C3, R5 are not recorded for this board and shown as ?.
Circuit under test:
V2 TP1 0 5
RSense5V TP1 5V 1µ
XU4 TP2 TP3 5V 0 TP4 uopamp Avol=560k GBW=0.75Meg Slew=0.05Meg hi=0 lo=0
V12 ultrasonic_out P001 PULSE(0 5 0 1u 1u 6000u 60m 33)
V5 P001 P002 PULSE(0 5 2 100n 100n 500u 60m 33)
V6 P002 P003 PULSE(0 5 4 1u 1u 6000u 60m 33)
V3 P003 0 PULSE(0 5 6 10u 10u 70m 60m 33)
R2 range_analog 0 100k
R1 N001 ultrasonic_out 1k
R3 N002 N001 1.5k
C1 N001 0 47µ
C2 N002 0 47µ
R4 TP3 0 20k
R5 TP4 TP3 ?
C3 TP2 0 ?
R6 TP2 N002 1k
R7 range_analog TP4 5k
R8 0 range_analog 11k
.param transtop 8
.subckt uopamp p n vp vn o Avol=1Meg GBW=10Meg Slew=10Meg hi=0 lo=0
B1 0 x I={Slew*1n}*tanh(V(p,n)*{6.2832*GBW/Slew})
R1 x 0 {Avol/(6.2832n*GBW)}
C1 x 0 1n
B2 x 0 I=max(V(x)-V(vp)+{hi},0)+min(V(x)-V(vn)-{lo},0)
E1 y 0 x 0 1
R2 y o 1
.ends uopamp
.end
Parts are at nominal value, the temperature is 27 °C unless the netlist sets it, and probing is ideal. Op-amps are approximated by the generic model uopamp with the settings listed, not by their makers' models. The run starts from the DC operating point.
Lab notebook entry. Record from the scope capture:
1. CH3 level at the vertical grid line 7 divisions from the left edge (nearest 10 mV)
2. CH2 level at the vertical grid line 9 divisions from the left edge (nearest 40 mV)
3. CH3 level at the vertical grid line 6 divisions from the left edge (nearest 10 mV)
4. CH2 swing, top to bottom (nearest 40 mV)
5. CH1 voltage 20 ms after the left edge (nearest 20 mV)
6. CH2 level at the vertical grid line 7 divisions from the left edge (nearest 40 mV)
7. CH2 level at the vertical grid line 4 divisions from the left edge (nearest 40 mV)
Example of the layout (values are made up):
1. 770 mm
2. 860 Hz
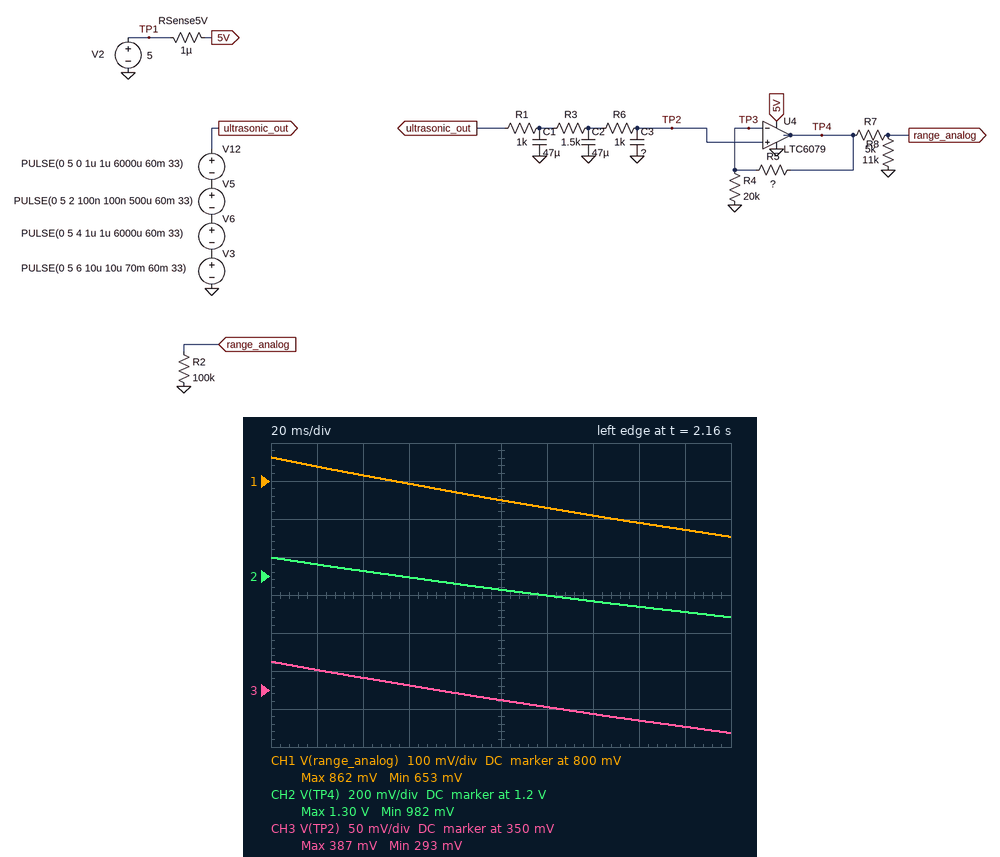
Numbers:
1. 320 mV
2. 1.00 V
3. 330 mV
4. 320 mV
5. 840 mV
6. 1.08 V
7. 1.16 V
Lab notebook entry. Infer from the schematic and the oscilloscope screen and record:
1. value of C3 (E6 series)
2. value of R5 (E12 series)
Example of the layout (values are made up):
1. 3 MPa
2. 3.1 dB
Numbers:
1. 150 µF
2. 47 kΩ
